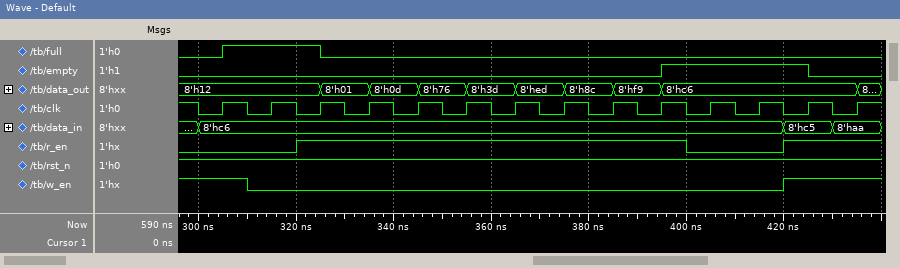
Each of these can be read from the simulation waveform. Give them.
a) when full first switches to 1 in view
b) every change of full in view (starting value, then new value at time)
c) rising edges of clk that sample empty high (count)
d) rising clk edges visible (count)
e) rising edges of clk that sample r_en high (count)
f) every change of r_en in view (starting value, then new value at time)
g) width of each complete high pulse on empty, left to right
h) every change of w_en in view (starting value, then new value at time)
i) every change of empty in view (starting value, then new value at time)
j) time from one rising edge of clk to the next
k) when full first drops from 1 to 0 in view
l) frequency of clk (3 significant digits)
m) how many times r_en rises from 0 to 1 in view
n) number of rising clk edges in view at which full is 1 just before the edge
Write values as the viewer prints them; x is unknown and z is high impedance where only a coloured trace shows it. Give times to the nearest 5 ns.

305 ns
0, 1 at 305 ns, 0 at 325 ns
3
14
10
0, 1 at 320 ns, 0 at 400 ns, 1 at 420 ns
30 ns
1, 0 at 310 ns, 1 at 420 ns
0, 1 at 395 ns, 0 at 425 ns
10 ns
325 ns
100 MHz
2
2
